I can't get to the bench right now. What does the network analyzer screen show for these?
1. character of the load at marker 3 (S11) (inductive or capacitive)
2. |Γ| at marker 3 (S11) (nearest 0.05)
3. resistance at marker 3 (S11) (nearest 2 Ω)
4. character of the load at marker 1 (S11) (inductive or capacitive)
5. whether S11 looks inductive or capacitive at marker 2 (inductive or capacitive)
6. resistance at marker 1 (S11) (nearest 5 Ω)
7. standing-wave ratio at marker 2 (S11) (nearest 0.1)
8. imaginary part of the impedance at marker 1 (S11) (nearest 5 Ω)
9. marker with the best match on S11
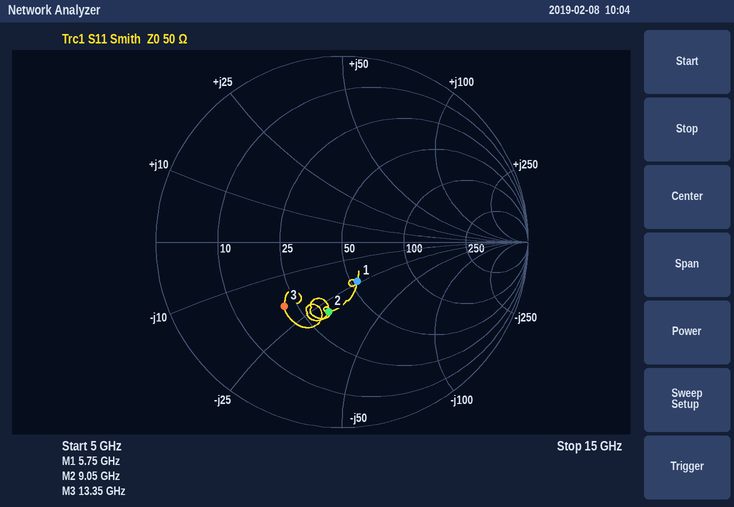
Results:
capacitive
0.45
22 Ω
capacitive
capacitive
55 Ω
2.2
-25 Ω
marker 1
